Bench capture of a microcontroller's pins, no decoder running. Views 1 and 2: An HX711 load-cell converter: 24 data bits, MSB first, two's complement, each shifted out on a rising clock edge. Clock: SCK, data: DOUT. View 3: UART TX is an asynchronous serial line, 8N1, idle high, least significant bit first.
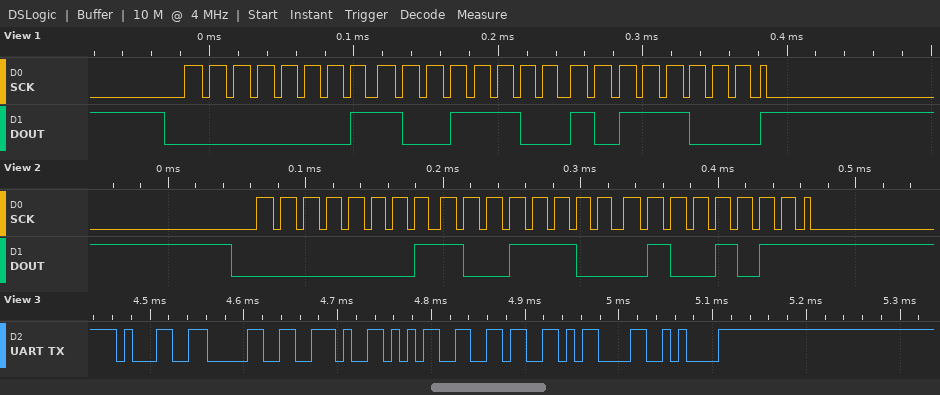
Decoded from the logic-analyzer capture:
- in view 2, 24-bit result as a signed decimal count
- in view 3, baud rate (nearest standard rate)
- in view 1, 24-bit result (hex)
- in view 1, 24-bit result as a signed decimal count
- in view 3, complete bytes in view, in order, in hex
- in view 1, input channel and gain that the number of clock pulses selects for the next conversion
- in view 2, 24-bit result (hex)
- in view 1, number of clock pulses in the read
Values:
105547
115200 baud
0x019CB8
105656
31 30 2E 35 36 0D 0A
channel A, gain 128
0x019C4B
25
